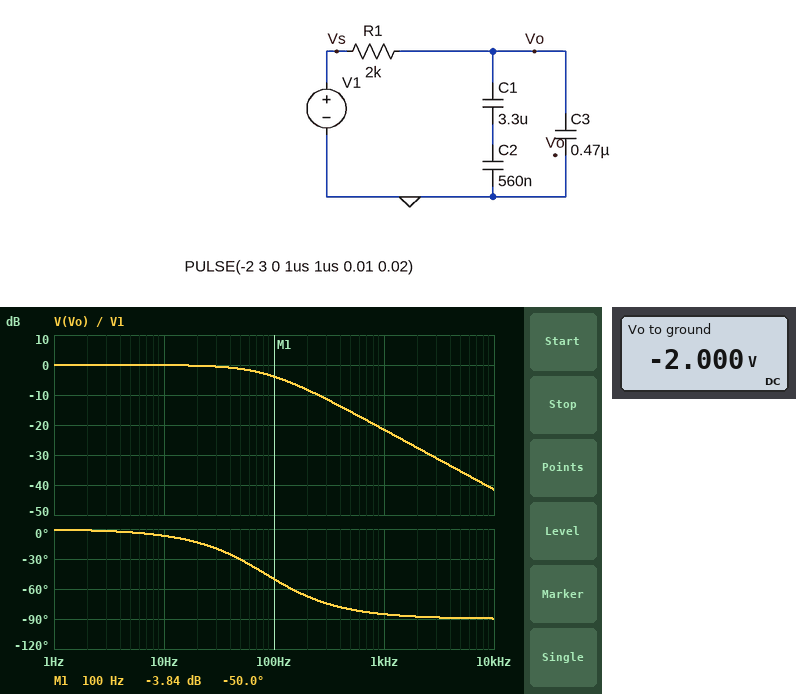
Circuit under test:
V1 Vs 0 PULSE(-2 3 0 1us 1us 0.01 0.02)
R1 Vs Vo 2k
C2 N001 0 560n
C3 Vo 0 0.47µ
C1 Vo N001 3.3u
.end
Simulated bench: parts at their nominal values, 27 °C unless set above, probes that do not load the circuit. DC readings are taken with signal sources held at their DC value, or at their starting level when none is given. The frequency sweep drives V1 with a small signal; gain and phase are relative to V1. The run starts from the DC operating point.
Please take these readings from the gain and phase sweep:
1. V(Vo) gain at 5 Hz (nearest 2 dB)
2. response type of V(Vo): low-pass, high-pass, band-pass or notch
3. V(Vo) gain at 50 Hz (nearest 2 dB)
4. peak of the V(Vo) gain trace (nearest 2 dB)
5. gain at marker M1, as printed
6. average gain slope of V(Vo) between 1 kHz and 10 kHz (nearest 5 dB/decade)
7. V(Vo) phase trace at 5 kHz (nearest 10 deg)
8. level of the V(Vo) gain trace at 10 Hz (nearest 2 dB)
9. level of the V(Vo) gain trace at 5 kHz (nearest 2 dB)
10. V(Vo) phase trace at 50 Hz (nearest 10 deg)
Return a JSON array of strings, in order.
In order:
["0 dB", "low-pass", "-2 dB", "0 dB", "-3.84 dB", "-20 dB/decade", "-90 deg", "0 dB", "-36 dB", "-30 deg"]
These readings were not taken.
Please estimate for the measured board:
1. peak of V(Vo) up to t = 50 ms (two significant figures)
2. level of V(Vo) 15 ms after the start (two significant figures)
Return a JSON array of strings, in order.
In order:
["3.0 V", "-1.6 V"]
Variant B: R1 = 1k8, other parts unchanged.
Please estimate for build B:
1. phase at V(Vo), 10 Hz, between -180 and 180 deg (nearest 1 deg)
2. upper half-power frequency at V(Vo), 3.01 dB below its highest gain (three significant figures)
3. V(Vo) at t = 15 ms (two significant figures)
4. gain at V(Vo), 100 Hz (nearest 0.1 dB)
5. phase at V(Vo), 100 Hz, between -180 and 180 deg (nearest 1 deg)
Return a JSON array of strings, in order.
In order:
["-6 deg", "93.2 Hz", "-1.7 V", "-3.3 dB", "-47 deg"]
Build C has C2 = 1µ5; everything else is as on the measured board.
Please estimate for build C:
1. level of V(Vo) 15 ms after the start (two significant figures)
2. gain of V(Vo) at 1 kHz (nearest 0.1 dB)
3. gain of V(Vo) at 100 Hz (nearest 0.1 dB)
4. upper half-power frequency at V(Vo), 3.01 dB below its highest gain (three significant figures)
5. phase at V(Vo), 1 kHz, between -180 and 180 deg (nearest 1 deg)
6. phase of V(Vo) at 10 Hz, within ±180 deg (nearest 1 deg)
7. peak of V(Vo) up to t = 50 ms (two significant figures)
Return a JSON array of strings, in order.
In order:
["-1.1 V", "-25.5 dB", "-6.6 dB", "53.0 Hz", "-87 deg", "-11 deg", "2.8 V"]
